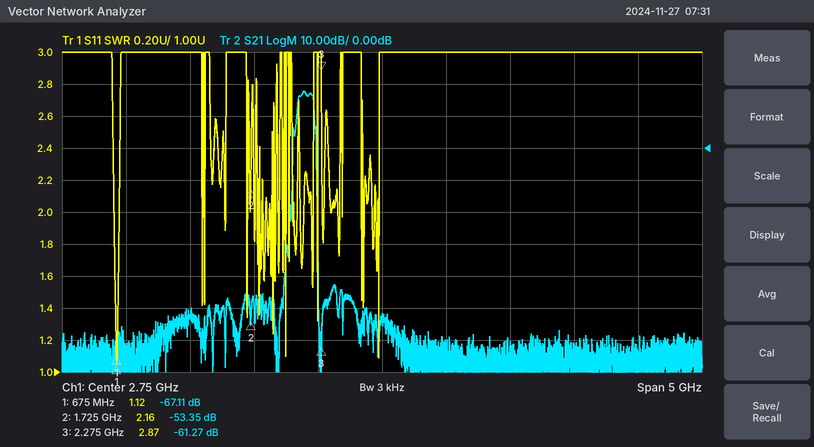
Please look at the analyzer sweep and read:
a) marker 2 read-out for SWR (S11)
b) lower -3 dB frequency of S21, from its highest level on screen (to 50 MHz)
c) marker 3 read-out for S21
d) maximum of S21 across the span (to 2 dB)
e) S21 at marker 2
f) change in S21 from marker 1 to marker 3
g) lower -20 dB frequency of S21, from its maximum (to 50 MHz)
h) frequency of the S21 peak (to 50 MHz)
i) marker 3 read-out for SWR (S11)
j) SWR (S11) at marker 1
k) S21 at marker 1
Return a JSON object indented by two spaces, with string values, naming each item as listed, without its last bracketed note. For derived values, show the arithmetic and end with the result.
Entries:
{
  "marker 2 read-out for SWR": "2.16",
  "lower -3 dB frequency of S21, from its highest level on screen": "2.10 GHz",
  "marker 3 read-out for S21": "-61.27 dB",
  "maximum of S21 across the span": "18 dB",
  "S21 at marker 2": "-53.35 dB",
  "change in S21 from marker 1 to marker 3": "-61.27 − (-67.11) = 5.84 dB",
  "lower -20 dB frequency of S21, from its maximum": "2.05 GHz",
  "frequency of the S21 peak": "2.15 GHz",
  "marker 3 read-out for SWR": "2.87",
  "SWR (S11) at marker 1": "1.12",
  "S21 at marker 1": "-67.11 dB"
}
